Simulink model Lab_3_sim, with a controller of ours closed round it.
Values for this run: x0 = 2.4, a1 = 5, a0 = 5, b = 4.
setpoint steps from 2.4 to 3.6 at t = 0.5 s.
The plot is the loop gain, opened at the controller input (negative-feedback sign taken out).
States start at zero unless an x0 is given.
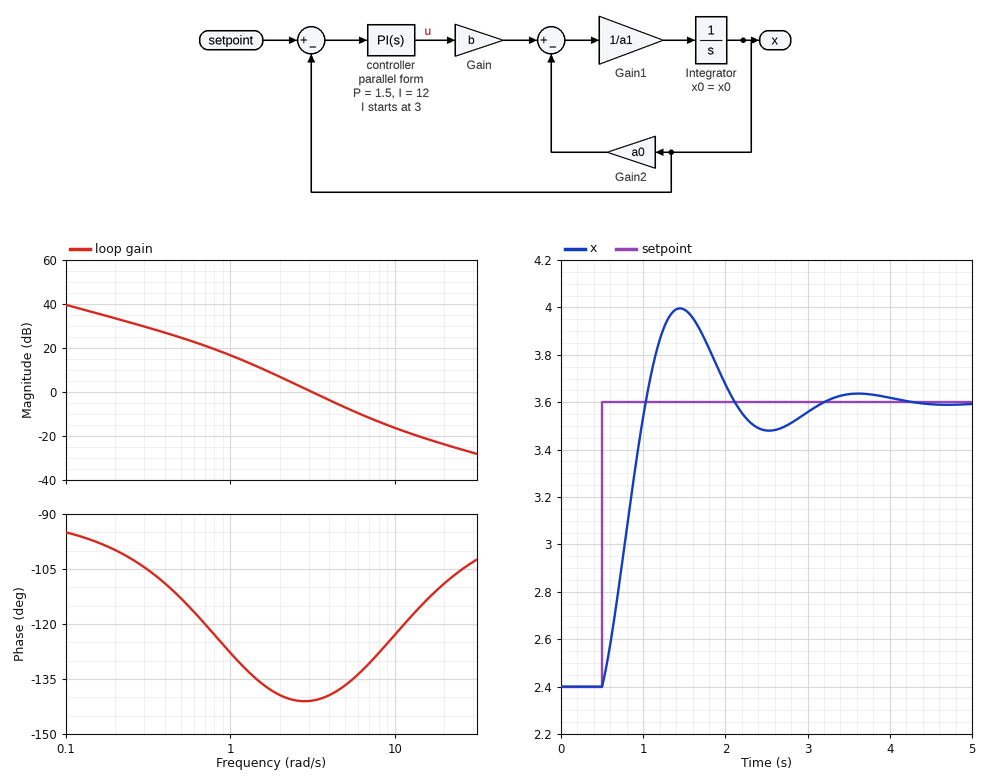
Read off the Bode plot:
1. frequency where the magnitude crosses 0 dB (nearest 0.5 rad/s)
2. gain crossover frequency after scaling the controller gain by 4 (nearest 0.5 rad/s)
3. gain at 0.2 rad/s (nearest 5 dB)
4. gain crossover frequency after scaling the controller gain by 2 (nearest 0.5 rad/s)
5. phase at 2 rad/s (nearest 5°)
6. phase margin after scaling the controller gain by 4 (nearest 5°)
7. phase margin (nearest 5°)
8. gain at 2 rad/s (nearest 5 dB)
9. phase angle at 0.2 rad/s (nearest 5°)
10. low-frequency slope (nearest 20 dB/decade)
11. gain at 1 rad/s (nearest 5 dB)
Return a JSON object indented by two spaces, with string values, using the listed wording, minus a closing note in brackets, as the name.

{
  "frequency where the magnitude crosses 0 dB": "3.0 rad/s",
  "gain crossover frequency after scaling the controller gain by 4": "7.0 rad/s",
  "gain at 0.2 rad/s": "35 dB",
  "gain crossover frequency after scaling the controller gain by 2": "4.5 rad/s",
  "phase at 2 rad/s": "-140°",
  "phase margin after scaling the controller gain by 4": "50°",
  "phase margin": "40°",
  "gain at 2 rad/s": "5 dB",
  "phase angle at 0.2 rad/s": "-100°",
  "low-frequency slope": "-20 dB/decade",
  "gain at 1 rad/s": "15 dB"
}
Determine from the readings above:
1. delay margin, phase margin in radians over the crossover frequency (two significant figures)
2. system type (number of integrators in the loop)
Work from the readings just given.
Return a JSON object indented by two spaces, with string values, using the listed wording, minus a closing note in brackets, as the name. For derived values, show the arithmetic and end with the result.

{
  "delay margin, phase margin in radians over the crossover frequency": "40 × π / 180 / 3 = 0.23 s",
  "system type": "1"
}
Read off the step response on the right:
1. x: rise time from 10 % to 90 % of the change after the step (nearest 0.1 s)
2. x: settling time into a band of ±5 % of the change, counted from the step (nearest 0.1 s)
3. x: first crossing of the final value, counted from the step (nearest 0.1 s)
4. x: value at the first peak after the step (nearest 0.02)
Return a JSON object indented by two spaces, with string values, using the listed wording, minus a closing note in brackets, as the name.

{
  "x: rise time from 10 % to 90 % of the change after the step": "0.4 s",
  "x: settling time into a band of ±5 % of the change, counted from the step": "2.4 s",
  "x: first crossing of the final value, counted from the step": "0.5 s",
  "x: value at the first peak after the step": "4.00"
}
